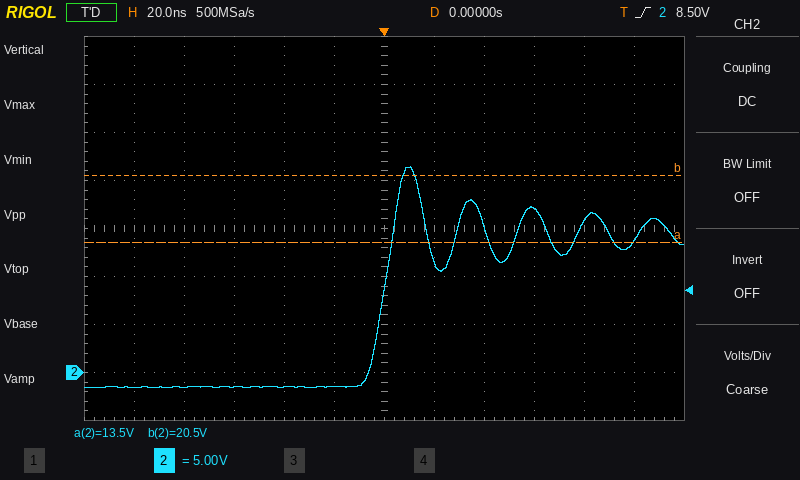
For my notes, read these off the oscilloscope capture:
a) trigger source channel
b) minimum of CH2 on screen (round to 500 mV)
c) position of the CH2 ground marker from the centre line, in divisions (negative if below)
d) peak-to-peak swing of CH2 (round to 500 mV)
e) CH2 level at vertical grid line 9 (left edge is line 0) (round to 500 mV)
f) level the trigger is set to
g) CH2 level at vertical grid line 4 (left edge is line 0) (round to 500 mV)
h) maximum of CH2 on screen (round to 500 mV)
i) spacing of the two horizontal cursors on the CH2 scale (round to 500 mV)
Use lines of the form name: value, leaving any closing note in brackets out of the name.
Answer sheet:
trigger source channel: CH2
minimum of CH2 on screen: -1.5 V
position of the CH2 ground marker from the centre line, in divisions: -3.0 div
peak-to-peak swing of CH2: 23.0 V
CH2 level at vertical grid line 9 (left edge is line 0): 17.0 V
level the trigger is set to: 8.50 V
CH2 level at vertical grid line 4 (left edge is line 0): -1.5 V
maximum of CH2 on screen: 21.5 V
spacing of the two horizontal cursors on the CH2 scale: 7.0 V
